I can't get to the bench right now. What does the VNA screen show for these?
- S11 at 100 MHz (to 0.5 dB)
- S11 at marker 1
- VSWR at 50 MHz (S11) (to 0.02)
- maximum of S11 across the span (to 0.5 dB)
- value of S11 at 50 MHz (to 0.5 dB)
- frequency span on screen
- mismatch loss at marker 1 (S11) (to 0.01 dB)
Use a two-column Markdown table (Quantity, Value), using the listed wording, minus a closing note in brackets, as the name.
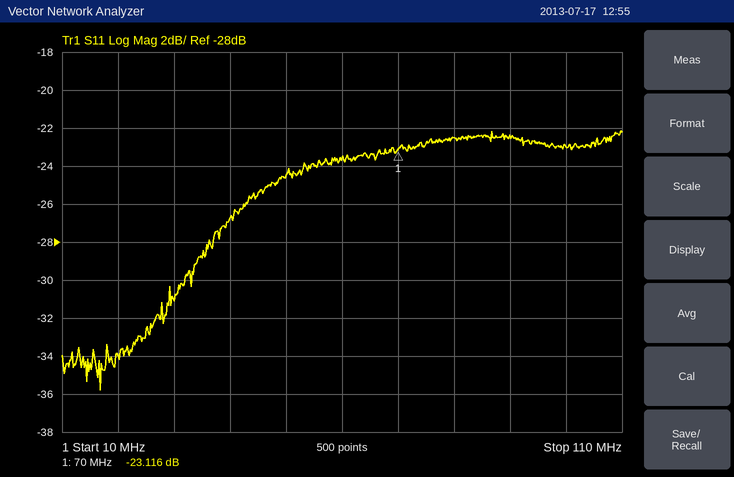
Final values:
| Quantity | Value |
|---|---|
| S11 at 100 MHz | -23.0 dB |
| S11 at marker 1 | -23.116 dB |
| VSWR at 50 MHz (S11) | 1.12 |
| maximum of S11 across the span | -22.0 dB |
| value of S11 at 50 MHz | -24.5 dB |
| frequency span on screen | 100 MHz |
| mismatch loss at marker 1 (S11) | 0.02 dB |
